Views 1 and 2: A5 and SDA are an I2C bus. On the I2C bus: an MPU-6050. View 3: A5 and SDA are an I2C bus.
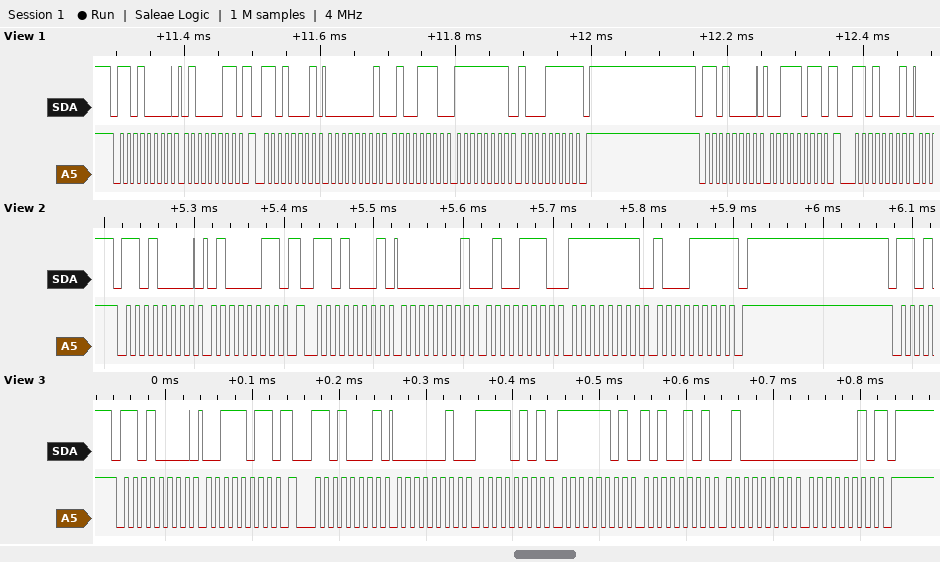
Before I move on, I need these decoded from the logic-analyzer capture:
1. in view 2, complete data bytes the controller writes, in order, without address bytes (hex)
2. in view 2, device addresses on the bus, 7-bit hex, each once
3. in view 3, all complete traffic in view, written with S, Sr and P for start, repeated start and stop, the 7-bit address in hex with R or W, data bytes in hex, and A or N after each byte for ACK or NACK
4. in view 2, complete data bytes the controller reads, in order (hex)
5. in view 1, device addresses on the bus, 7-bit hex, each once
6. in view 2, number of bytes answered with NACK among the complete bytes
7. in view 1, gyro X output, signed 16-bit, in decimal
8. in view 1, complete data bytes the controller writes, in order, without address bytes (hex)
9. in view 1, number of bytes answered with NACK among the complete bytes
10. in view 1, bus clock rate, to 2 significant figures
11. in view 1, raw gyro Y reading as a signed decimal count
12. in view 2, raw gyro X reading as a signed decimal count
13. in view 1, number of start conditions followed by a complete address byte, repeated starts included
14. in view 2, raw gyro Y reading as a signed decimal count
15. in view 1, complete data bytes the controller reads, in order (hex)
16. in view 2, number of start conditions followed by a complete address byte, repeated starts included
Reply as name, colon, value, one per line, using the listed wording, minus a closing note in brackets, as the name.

in view 2, complete data bytes the controller writes, in order, without address bytes: 43
in view 2, device addresses on the bus, 7-bit hex, each once: 0x68
in view 3, all complete traffic in view, written with S, Sr and P for start, repeated start and stop, the 7-bit address in hex with R or W, data bytes in hex, and A or N after each byte for ACK or NACK: S 68W A 3B A Sr 68R A 02 A F5 A FD A A5 A 40 A 02 N P
in view 2, complete data bytes the controller reads, in order: 01 4E FF 8F
in view 1, device addresses on the bus, 7-bit hex, each once: 0x68
in view 2, number of bytes answered with NACK among the complete bytes: 1
in view 1, gyro X output, signed 16-bit, in decimal: 334
in view 1, complete data bytes the controller writes, in order, without address bytes: 43 3B
in view 1, number of bytes answered with NACK among the complete bytes: 1
in view 1, bus clock rate, to 2 significant figures: 100 kHz
in view 1, raw gyro Y reading as a signed decimal count: -113
in view 2, raw gyro X reading as a signed decimal count: 334
in view 1, number of start conditions followed by a complete address byte, repeated starts included: 4
in view 2, raw gyro Y reading as a signed decimal count: -113
in view 1, complete data bytes the controller reads, in order: 01 4E FF 8F
in view 2, number of start conditions followed by a complete address byte, repeated starts included: 2
